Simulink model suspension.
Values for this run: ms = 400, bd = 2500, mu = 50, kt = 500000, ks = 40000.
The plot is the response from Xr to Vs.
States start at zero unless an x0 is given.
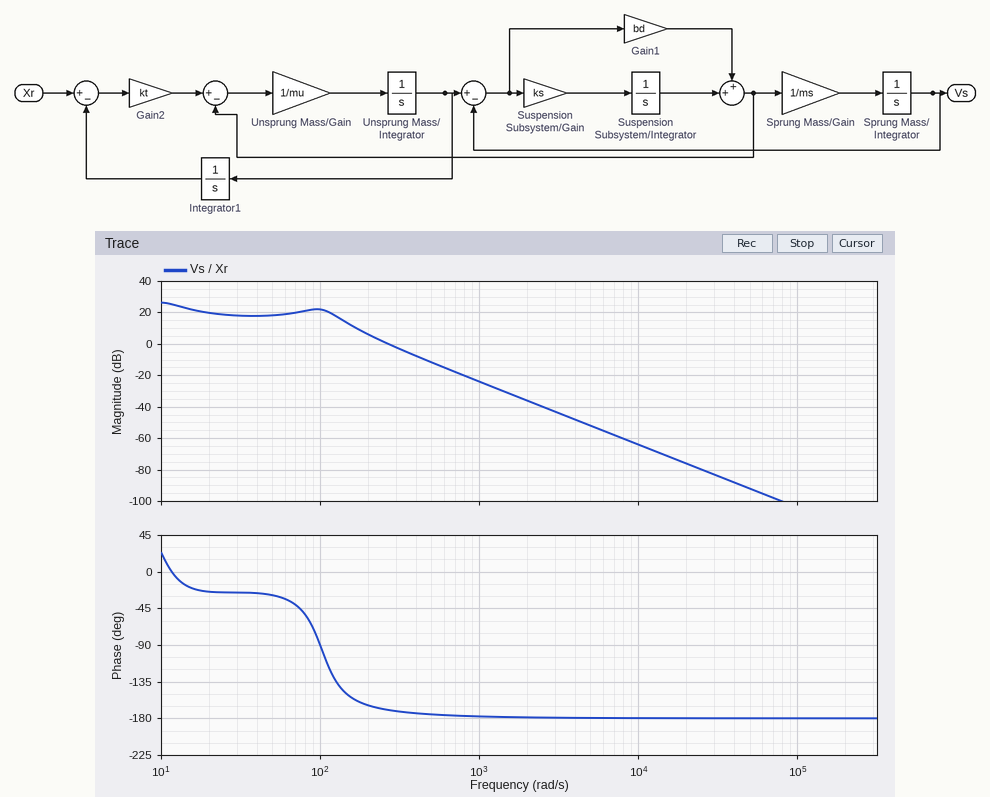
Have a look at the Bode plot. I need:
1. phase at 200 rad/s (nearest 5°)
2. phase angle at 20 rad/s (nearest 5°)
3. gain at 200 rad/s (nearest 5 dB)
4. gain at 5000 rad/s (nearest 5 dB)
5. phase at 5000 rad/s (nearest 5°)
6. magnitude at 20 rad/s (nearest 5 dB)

-165°
-25°
5 dB
-50 dB
-180°
20 dB
